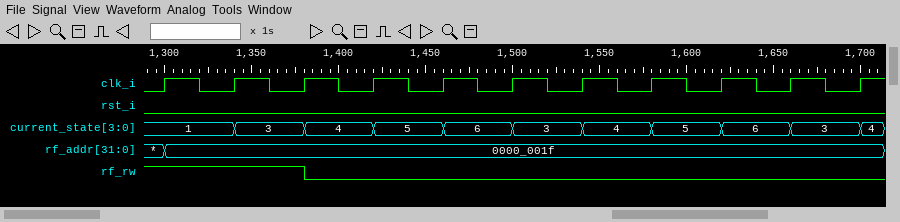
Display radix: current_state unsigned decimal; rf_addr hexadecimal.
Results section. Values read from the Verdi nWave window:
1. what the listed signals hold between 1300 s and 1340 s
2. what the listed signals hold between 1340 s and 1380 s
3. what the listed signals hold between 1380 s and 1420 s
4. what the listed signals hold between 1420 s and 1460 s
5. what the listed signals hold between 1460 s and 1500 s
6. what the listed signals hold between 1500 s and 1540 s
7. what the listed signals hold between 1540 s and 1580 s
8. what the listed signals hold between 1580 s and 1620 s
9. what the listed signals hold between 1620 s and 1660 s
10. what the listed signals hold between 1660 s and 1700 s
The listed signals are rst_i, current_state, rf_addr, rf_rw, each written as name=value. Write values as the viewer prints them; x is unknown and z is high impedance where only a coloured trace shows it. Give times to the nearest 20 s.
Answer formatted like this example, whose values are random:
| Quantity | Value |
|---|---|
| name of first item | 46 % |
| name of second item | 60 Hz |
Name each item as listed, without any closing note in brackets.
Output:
| Quantity | Value |
|---|---|
| what the listed signals hold between 1300 s and 1340 s | rst_i=0, current_state=1, rf_addr=0000_001f, rf_rw=1 |
| what the listed signals hold between 1340 s and 1380 s | rst_i=0, current_state=3, rf_addr=0000_001f, rf_rw=1 |
| what the listed signals hold between 1380 s and 1420 s | rst_i=0, current_state=4, rf_addr=0000_001f, rf_rw=0 |
| what the listed signals hold between 1420 s and 1460 s | rst_i=0, current_state=5, rf_addr=0000_001f, rf_rw=0 |
| what the listed signals hold between 1460 s and 1500 s | rst_i=0, current_state=6, rf_addr=0000_001f, rf_rw=0 |
| what the listed signals hold between 1500 s and 1540 s | rst_i=0, current_state=3, rf_addr=0000_001f, rf_rw=0 |
| what the listed signals hold between 1540 s and 1580 s | rst_i=0, current_state=4, rf_addr=0000_001f, rf_rw=0 |
| what the listed signals hold between 1580 s and 1620 s | rst_i=0, current_state=5, rf_addr=0000_001f, rf_rw=0 |
| what the listed signals hold between 1620 s and 1660 s | rst_i=0, current_state=6, rf_addr=0000_001f, rf_rw=0 |
| what the listed signals hold between 1660 s and 1700 s | rst_i=0, current_state=3, rf_addr=0000_001f, rf_rw=0 |
